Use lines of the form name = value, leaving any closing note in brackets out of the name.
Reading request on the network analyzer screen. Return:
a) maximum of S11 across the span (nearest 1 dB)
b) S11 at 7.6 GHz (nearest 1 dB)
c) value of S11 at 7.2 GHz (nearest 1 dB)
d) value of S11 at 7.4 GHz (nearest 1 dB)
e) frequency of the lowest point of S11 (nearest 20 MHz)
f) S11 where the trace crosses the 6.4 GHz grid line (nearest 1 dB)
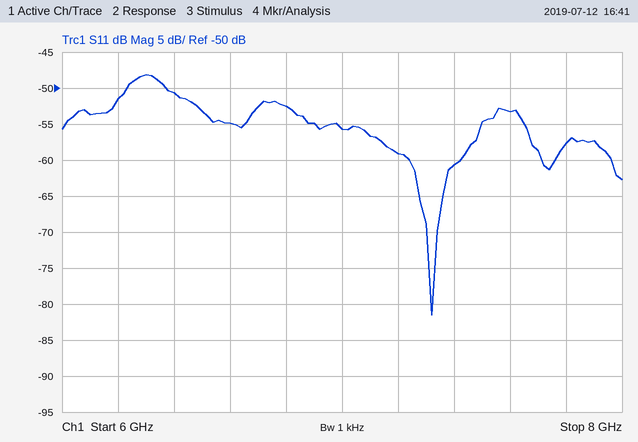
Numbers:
maximum of S11 across the span = -48 dB
S11 at 7.6 GHz = -53 dB
value of S11 at 7.2 GHz = -59 dB
value of S11 at 7.4 GHz = -61 dB
frequency of the lowest point of S11 = 7.32 GHz
S11 where the trace crosses the 6.4 GHz grid line = -51 dB
